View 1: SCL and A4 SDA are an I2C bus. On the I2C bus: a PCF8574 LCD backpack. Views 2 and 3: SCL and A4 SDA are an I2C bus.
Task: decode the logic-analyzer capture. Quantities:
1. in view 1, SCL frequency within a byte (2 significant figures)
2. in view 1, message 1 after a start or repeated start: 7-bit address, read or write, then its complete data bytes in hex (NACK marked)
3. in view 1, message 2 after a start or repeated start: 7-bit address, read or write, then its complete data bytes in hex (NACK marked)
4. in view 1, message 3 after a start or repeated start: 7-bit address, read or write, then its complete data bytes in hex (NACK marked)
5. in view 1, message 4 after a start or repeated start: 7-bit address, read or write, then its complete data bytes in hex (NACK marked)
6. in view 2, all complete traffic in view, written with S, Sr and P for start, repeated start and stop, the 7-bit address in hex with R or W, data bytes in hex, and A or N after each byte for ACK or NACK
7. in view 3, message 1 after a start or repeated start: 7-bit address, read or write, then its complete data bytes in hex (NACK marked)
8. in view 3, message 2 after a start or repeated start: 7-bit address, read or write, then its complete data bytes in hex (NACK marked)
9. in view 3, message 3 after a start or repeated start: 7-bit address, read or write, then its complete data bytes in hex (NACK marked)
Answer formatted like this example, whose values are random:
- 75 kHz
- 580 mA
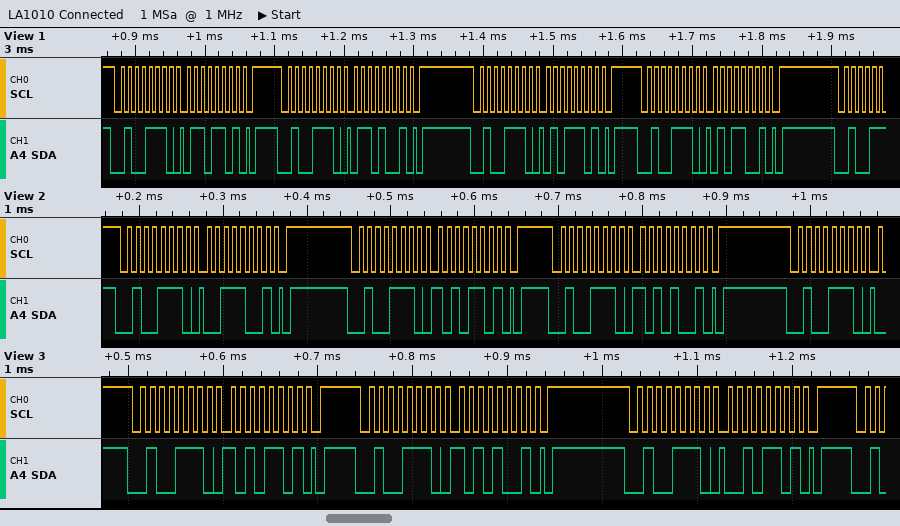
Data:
- 100 kHz
- 0x27 write: 6D
- 0x27 write: 69
- 0x27 write: 5D
- 0x27 write: 59
- S 27W A 39 A P S 27W A AD A P S 27W A A9 A P S 27W A
- 0x27 write: AD
- 0x27 write: A9
- 0x27 write: 2D
